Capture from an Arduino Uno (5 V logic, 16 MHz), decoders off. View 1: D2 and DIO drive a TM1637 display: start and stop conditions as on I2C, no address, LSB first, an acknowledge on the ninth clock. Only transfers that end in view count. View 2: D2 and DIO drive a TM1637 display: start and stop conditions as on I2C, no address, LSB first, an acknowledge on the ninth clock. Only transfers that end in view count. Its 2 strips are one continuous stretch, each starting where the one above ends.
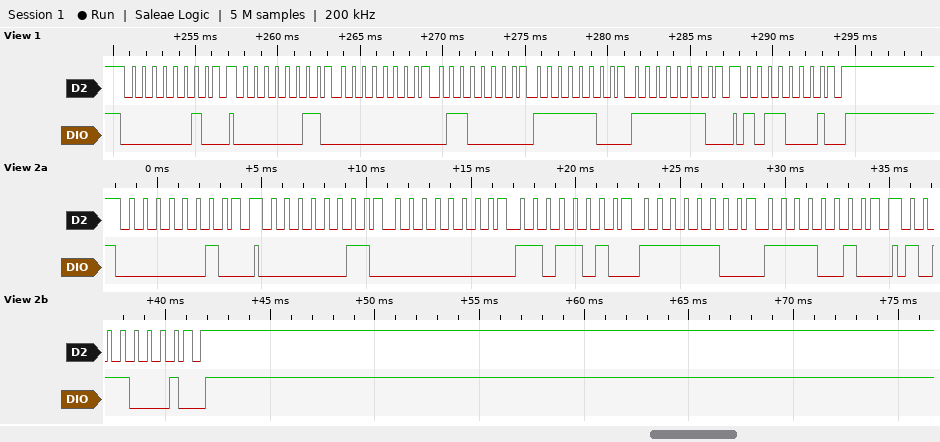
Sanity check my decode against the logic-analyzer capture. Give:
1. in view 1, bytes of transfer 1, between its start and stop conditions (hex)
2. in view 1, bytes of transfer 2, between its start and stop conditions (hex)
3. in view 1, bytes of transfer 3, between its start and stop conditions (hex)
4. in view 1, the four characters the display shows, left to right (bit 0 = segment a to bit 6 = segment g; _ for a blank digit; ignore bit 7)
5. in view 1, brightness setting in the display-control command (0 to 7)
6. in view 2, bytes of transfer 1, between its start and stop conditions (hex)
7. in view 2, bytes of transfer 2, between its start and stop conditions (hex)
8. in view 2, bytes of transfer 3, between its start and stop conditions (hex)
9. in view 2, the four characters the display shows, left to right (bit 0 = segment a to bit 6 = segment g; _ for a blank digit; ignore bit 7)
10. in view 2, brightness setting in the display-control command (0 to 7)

40
C0 00 06 3F 7F
8D
_108
5
40
C0 00 5B 3F 4F
8D
_203
5
